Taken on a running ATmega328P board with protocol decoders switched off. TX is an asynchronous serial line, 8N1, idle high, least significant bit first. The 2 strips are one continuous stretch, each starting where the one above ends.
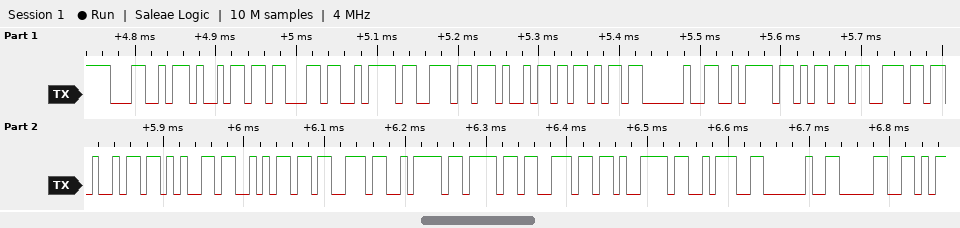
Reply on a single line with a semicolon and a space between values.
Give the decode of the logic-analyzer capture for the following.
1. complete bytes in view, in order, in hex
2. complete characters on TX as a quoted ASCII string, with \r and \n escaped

4C 69 63 7A 6E 69 6B 20 7A 6D 6E 69 65 6A 73 7A 6F 6E 79 3A 20 30; "Licznik zmniejszony: 0"
